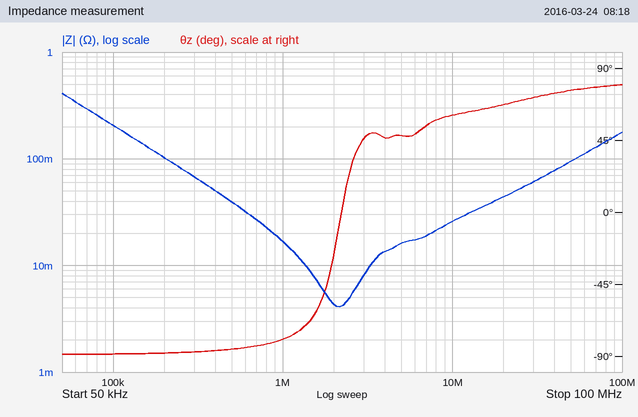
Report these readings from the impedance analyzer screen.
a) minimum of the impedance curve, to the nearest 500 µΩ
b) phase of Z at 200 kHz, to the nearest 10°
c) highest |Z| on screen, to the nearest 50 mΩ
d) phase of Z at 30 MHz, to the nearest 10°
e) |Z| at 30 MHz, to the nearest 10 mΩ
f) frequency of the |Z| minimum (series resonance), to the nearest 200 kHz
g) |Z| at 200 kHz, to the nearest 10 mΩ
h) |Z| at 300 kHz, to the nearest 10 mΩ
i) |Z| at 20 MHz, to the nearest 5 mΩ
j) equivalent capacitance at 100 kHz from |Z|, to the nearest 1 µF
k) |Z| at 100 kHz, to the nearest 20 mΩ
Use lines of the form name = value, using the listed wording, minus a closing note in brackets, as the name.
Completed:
minimum of the impedance curve, to the nearest 500 µΩ = 4.0 mΩ
phase of Z at 200 kHz, to the nearest 10° = -90°
highest |Z| on screen, to the nearest 50 mΩ = 400 mΩ
phase of Z at 30 MHz, to the nearest 10° = 70°
|Z| at 30 MHz, to the nearest 10 mΩ = 60 mΩ
frequency of the |Z| minimum (series resonance), to the nearest 200 kHz = 2.2 MHz
|Z| at 200 kHz, to the nearest 10 mΩ = 100 mΩ
|Z| at 300 kHz, to the nearest 10 mΩ = 70 mΩ
|Z| at 20 MHz, to the nearest 5 mΩ = 45 mΩ
equivalent capacitance at 100 kHz from |Z|, to the nearest 1 µF = 8 µF
|Z| at 100 kHz, to the nearest 20 mΩ = 200 mΩ
